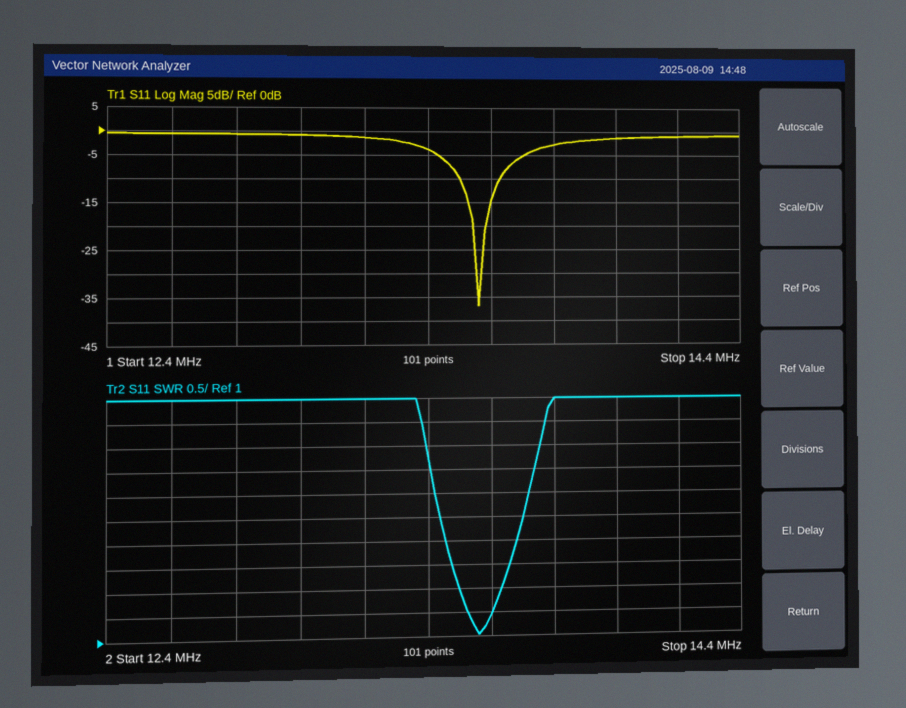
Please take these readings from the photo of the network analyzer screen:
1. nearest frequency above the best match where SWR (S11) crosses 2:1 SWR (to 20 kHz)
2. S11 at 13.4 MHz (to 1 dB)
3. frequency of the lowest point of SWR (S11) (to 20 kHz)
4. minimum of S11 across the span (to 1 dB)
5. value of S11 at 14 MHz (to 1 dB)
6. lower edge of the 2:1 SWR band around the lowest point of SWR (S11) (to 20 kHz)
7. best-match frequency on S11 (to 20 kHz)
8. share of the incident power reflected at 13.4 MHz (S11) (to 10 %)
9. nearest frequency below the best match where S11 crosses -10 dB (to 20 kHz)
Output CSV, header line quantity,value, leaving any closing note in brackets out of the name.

quantity,value
nearest frequency above the best match where SWR (S11) crosses 2:1 SWR,13.64 MHz
S11 at 13.4 MHz,-4 dB
frequency of the lowest point of SWR (S11),13.56 MHz
minimum of S11 across the span,-37 dB
value of S11 at 14 MHz,-1 dB
lower edge of the 2:1 SWR band around the lowest point of SWR (S11),13.50 MHz
best-match frequency on S11,13.56 MHz
share of the incident power reflected at 13.4 MHz (S11),40 %
nearest frequency below the best match where S11 crosses -10 dB,13.50 MHz
